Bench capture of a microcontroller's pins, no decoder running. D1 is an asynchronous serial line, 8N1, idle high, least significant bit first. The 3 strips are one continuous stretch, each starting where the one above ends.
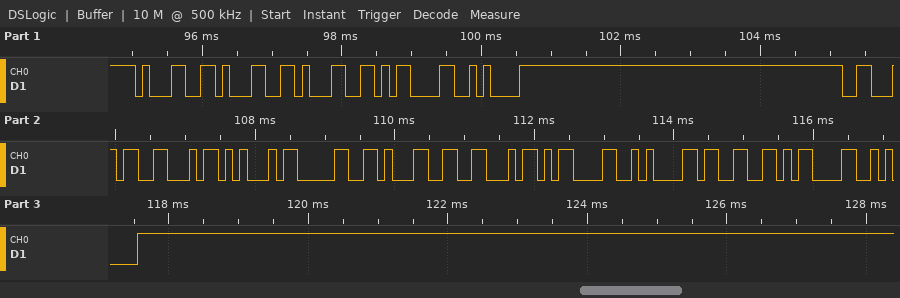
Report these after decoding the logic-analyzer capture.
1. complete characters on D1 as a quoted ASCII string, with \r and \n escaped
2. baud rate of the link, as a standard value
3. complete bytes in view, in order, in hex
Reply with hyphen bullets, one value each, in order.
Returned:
- "111\r\nFFE01F\r\n3\r\n"
- 9600 baud
- 31 31 31 0D 0A 46 46 45 30 31 46 0D 0A 33 0D 0A
